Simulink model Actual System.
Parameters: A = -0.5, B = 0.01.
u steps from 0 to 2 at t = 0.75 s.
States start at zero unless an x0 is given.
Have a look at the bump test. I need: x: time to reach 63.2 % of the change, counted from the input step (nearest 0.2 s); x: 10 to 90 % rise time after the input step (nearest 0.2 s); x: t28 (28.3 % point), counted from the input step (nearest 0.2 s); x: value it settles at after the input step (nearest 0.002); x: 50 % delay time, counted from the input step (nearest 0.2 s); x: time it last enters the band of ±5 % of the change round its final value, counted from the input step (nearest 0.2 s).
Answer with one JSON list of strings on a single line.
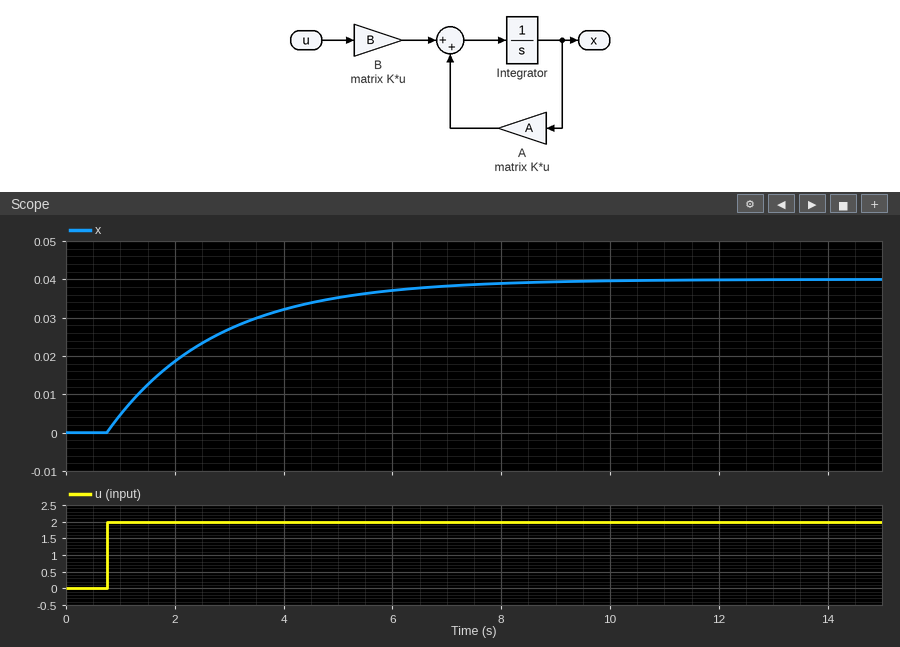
["2.0 s", "4.4 s", "0.6 s", "0.040", "1.4 s", "6.0 s"]
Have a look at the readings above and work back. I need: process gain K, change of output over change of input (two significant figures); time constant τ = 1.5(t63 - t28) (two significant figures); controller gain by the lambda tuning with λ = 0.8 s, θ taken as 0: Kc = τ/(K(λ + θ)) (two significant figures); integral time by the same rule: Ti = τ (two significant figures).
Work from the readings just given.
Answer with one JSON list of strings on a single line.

["0.020", "2.1 s", "130", "2.1 s"]
